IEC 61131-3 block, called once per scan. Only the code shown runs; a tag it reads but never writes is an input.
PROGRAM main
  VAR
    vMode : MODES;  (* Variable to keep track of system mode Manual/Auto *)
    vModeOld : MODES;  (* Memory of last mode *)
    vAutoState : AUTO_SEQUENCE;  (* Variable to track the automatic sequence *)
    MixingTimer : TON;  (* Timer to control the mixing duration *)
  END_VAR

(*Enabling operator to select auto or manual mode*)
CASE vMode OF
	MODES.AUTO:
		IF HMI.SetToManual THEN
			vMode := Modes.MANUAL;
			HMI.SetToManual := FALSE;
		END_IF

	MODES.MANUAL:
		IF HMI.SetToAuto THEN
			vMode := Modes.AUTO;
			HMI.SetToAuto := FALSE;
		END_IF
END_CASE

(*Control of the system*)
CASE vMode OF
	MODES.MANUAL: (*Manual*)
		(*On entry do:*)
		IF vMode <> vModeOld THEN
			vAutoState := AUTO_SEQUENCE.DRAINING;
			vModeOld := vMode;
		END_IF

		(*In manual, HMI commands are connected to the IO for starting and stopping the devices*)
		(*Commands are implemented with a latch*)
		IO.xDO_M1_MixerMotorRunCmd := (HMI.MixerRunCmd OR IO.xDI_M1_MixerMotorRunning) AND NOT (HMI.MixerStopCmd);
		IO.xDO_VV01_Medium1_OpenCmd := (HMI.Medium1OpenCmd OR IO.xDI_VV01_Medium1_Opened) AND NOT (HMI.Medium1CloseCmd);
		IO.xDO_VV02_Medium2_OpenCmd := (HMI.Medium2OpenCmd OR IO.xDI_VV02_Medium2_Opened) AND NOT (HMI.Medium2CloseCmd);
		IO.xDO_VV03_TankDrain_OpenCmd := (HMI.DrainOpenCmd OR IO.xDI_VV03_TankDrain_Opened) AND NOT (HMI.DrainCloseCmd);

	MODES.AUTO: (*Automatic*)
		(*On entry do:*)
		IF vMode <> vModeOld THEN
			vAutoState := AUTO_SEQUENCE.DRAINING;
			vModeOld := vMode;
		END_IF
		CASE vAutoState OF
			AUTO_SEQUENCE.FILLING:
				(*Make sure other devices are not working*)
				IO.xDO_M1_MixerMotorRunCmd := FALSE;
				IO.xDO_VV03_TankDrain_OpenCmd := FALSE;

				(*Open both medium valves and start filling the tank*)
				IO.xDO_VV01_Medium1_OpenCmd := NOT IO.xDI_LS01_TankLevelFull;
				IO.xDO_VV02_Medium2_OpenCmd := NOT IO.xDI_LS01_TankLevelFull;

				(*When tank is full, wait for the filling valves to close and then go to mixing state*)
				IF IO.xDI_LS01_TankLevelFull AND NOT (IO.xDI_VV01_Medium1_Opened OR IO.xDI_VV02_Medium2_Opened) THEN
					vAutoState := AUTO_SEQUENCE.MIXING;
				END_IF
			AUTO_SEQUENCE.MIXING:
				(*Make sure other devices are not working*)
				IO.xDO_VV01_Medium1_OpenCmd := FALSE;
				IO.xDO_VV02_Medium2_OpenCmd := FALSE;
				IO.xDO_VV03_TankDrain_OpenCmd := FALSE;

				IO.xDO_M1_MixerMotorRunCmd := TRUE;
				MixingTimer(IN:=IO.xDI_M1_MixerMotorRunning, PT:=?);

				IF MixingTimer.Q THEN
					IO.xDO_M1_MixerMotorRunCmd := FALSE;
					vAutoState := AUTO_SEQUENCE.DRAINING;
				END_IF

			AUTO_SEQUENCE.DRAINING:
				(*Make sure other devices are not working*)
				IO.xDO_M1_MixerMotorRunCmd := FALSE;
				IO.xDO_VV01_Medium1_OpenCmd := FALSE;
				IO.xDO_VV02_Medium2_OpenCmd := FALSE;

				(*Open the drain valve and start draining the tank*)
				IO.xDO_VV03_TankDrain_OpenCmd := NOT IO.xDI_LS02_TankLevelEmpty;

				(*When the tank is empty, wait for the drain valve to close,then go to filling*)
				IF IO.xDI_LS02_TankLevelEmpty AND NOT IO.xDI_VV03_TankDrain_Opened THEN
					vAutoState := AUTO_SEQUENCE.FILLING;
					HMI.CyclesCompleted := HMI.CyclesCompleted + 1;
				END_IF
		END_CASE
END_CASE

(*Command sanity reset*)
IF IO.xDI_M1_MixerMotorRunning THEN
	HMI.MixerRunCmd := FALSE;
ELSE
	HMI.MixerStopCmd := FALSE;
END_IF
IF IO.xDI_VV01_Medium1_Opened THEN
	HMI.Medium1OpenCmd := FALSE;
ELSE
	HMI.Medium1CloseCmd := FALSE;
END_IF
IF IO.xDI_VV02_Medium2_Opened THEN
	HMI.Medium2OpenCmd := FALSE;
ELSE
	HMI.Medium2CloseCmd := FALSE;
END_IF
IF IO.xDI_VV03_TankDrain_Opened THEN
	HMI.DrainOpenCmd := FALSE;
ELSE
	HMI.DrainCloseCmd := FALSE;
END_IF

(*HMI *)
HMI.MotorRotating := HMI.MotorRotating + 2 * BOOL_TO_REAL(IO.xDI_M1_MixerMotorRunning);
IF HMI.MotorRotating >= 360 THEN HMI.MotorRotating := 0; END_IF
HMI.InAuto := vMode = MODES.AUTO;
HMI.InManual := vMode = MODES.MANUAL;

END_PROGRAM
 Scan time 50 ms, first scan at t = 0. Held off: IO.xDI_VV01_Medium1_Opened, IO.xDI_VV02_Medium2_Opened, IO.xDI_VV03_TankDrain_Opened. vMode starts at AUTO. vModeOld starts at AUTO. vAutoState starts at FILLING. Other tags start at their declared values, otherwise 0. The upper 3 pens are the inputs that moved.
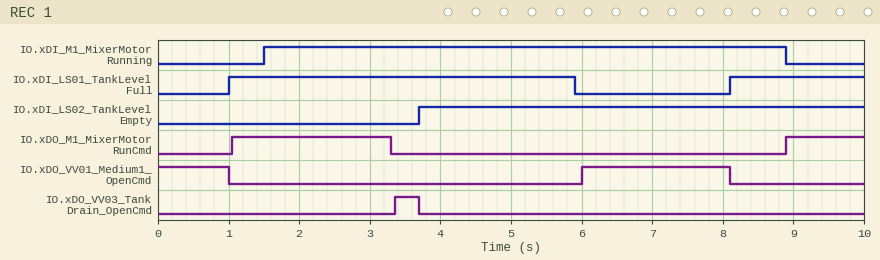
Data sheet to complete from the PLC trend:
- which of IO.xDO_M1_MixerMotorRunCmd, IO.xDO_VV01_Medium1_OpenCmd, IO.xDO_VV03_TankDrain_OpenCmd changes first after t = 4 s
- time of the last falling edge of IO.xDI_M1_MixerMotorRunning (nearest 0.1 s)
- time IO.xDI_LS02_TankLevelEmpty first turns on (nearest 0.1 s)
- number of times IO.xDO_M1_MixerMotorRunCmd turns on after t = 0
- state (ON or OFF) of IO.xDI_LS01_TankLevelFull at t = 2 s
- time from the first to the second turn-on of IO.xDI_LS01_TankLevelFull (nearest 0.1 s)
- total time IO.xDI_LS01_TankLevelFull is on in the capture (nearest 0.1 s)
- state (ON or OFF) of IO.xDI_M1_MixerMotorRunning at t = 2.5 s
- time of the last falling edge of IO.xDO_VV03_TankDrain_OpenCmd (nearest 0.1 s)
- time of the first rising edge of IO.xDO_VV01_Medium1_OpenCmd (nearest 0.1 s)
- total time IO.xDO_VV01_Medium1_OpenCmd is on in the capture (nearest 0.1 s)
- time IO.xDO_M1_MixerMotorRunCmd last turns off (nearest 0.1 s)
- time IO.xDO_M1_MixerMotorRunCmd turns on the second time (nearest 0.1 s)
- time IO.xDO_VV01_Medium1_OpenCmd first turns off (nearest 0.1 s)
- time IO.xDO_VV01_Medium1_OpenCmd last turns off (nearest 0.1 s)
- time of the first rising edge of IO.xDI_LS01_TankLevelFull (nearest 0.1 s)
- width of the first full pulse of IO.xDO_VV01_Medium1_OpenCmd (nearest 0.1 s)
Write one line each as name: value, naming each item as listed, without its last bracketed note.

which of IO.xDO_M1_MixerMotorRunCmd, IO.xDO_VV01_Medium1_OpenCmd, IO.xDO_VV03_TankDrain_OpenCmd changes first after t = 4 s: IO.xDO_VV01_Medium1_OpenCmd
time of the last falling edge of IO.xDI_M1_MixerMotorRunning: 8.9 s
time IO.xDI_LS02_TankLevelEmpty first turns on: 3.7 s
number of times IO.xDO_M1_MixerMotorRunCmd turns on after t = 0: 2
state (ON or OFF) of IO.xDI_LS01_TankLevelFull at t = 2 s: ON
time from the first to the second turn-on of IO.xDI_LS01_TankLevelFull: 7.1 s
total time IO.xDI_LS01_TankLevelFull is on in the capture: 6.8 s
state (ON or OFF) of IO.xDI_M1_MixerMotorRunning at t = 2.5 s: ON
time of the last falling edge of IO.xDO_VV03_TankDrain_OpenCmd: 3.7 s
time of the first rising edge of IO.xDO_VV01_Medium1_OpenCmd: 6.0 s
total time IO.xDO_VV01_Medium1_OpenCmd is on in the capture: 3.1 s
time IO.xDO_M1_MixerMotorRunCmd last turns off: 3.3 s
time IO.xDO_M1_MixerMotorRunCmd turns on the second time: 8.9 s
time IO.xDO_VV01_Medium1_OpenCmd first turns off: 1.0 s
time IO.xDO_VV01_Medium1_OpenCmd last turns off: 8.1 s
time of the first rising edge of IO.xDI_LS01_TankLevelFull: 1.0 s
width of the first full pulse of IO.xDO_VV01_Medium1_OpenCmd: 2.1 s
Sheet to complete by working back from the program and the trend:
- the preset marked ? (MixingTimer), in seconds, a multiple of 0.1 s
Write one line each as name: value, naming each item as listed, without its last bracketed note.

the preset marked ? (MixingTimer), in seconds, a multiple of 0.1 s: 1.8 s
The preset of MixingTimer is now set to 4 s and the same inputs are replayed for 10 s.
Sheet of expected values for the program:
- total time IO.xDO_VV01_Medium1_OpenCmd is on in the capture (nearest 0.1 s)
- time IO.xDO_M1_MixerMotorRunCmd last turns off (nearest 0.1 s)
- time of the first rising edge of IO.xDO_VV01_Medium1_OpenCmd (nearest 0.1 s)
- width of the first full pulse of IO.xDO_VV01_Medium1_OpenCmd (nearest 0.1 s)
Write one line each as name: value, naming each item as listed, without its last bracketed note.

total time IO.xDO_VV01_Medium1_OpenCmd is on in the capture: 3.2 s
time IO.xDO_M1_MixerMotorRunCmd last turns off: 5.5 s
time of the first rising edge of IO.xDO_VV01_Medium1_OpenCmd: 5.9 s
width of the first full pulse of IO.xDO_VV01_Medium1_OpenCmd: 2.2 s
